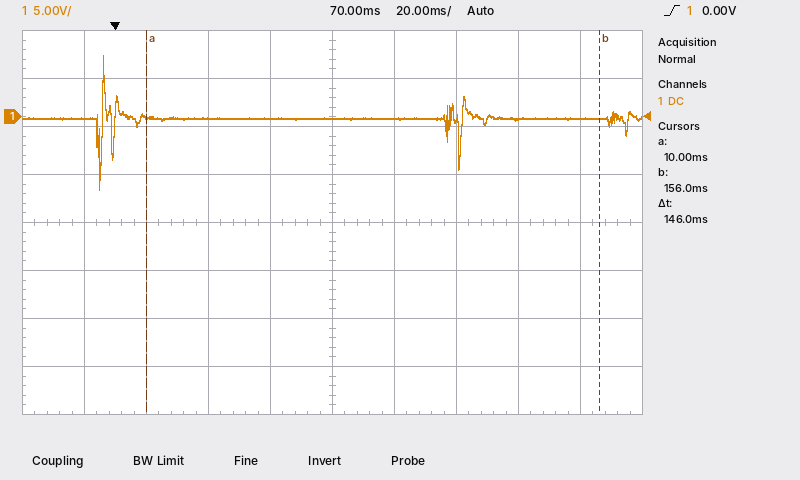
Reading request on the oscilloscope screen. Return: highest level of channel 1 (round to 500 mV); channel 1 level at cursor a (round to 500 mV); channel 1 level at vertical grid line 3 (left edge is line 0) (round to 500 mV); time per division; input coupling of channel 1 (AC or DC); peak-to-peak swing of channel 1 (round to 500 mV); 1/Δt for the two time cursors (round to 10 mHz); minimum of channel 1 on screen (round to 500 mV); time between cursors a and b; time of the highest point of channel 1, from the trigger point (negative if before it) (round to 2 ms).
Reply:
6.5 V
0.0 V
0.0 V
20 ms
DC
14.0 V
6.85 Hz
-7.5 V
146 ms
-4 ms
